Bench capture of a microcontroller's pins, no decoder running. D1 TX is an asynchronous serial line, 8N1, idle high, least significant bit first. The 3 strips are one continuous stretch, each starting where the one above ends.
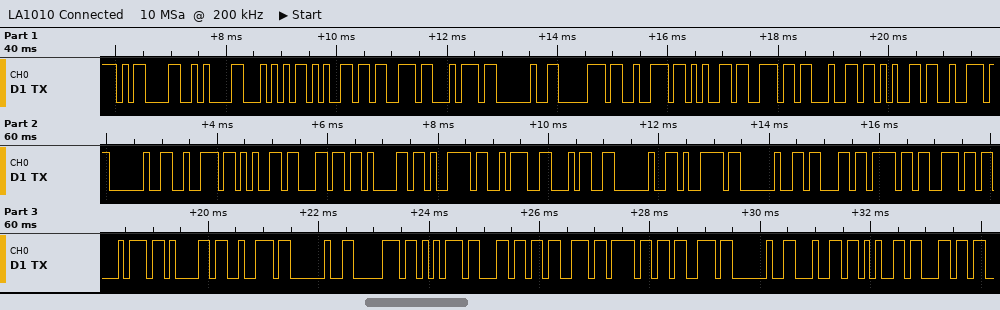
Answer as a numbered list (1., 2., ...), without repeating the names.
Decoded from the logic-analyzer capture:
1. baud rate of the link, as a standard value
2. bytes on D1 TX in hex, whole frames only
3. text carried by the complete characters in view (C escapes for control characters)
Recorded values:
1. 9600 baud
2. 0D 0A 54 65 73 74 20 70 72 65 6E 64 65 72 20 72 65 6C 61 79 3A 34 20 79 20 63 6F 6E 74 61 72 20 70 75 6C 73 6F 73 20 64 65 6C
3. "\r\nTest prender relay:4 y contar pulsos del"
